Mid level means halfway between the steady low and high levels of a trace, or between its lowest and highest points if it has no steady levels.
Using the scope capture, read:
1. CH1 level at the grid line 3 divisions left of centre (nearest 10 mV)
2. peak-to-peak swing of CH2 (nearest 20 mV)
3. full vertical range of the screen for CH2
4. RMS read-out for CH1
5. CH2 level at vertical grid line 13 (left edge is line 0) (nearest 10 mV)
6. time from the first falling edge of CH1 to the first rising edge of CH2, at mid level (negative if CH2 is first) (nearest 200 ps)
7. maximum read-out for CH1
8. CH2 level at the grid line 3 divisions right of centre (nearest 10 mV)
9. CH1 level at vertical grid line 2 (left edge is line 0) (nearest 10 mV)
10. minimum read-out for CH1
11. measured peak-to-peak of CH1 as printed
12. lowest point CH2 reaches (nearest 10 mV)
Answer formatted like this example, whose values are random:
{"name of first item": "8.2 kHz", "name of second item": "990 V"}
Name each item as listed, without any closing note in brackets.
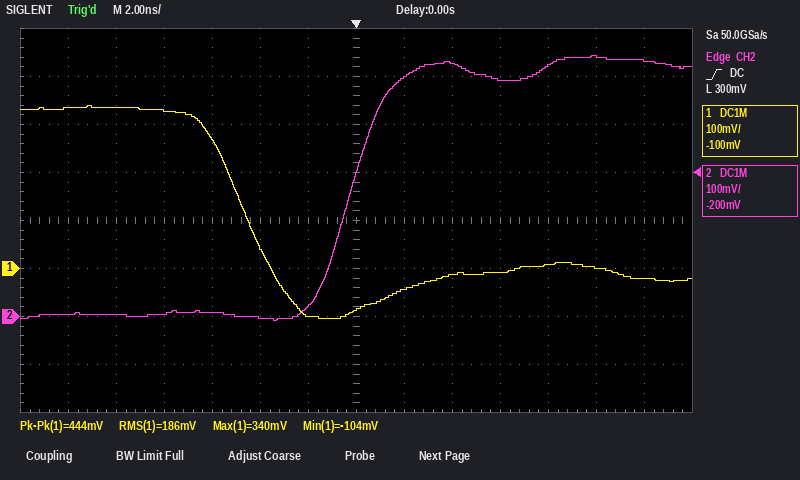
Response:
{"CH1 level at the grid line 3 divisions left of centre": "270 mV", "peak-to-peak swing of CH2": "560 mV", "full vertical range of the screen for CH2": "800 mV", "RMS read-out for CH1": "186 mV", "CH2 level at vertical grid line 13 (left edge is line 0)": "530 mV", "time from the first falling edge of CH1 to the first rising edge of CH2, at mid level (negative if CH2 is first)": "+4.4 ns", "maximum read-out for CH1": "340 mV", "CH2 level at the grid line 3 divisions right of centre": "490 mV", "CH1 level at vertical grid line 2 (left edge is line 0)": "340 mV", "minimum read-out for CH1": "-104 mV", "measured peak-to-peak of CH1 as printed": "444 mV", "lowest point CH2 reaches": "-10 mV"}
